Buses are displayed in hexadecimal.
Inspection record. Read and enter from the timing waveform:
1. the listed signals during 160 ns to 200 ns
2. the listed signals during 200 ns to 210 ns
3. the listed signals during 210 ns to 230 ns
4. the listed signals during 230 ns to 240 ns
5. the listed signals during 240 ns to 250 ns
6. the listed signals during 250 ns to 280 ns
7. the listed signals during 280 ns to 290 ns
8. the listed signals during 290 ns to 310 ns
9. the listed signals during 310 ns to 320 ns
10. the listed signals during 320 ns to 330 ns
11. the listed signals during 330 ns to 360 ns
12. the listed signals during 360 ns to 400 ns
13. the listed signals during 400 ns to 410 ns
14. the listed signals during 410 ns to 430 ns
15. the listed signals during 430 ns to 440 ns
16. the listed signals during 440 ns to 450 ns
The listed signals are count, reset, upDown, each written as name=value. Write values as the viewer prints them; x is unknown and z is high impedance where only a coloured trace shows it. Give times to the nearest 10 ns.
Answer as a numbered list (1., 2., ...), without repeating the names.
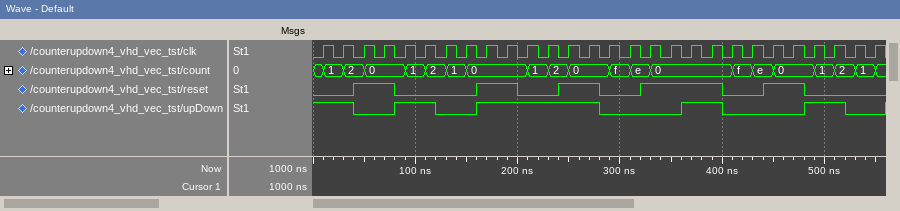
1. count=0, reset=1, upDown=1
2. count=0, reset=0, upDown=1
3. count=1, reset=0, upDown=1
4. count=2, reset=0, upDown=1
5. count=2, reset=1, upDown=1
6. count=0, reset=1, upDown=1
7. count=0, reset=0, upDown=0
8. count=f, reset=0, upDown=0
9. count=e, reset=0, upDown=0
10. count=e, reset=1, upDown=0
11. count=0, reset=1, upDown=0
12. count=0, reset=1, upDown=1
13. count=0, reset=0, upDown=0
14. count=f, reset=0, upDown=0
15. count=e, reset=0, upDown=0
16. count=e, reset=1, upDown=0
